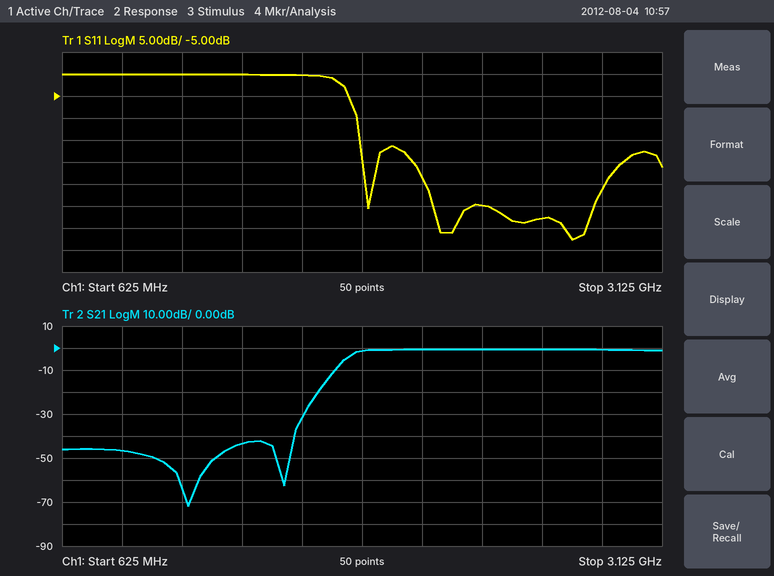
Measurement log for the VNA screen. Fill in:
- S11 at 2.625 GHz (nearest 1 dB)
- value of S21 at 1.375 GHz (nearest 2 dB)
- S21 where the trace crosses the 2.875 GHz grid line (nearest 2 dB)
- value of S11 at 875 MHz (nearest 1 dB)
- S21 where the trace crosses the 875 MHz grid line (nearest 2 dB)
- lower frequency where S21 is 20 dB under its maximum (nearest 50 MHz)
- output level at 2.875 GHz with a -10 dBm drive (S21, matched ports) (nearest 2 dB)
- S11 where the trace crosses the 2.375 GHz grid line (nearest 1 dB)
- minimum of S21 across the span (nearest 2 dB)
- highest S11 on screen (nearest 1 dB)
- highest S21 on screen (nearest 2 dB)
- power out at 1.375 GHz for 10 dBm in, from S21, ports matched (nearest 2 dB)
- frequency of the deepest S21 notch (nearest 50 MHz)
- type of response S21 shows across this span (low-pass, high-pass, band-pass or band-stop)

-33 dB
-44 dB
0 dB
0 dB
-46 dB
1.70 GHz
-10 dBm
-30 dB
-72 dB
0 dB
0 dB
-34 dBm
1.15 GHz
high-pass
